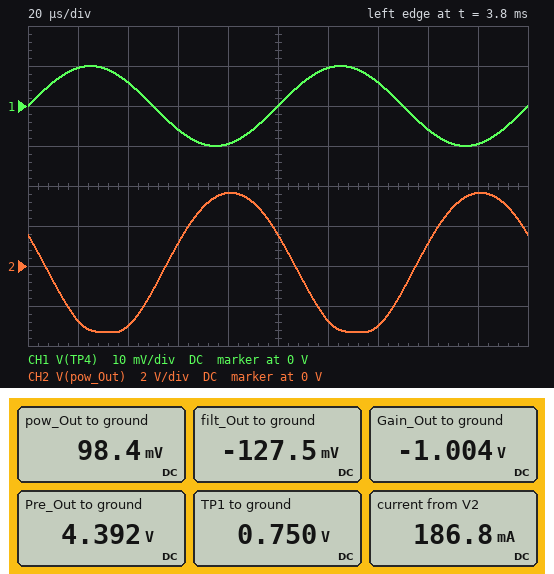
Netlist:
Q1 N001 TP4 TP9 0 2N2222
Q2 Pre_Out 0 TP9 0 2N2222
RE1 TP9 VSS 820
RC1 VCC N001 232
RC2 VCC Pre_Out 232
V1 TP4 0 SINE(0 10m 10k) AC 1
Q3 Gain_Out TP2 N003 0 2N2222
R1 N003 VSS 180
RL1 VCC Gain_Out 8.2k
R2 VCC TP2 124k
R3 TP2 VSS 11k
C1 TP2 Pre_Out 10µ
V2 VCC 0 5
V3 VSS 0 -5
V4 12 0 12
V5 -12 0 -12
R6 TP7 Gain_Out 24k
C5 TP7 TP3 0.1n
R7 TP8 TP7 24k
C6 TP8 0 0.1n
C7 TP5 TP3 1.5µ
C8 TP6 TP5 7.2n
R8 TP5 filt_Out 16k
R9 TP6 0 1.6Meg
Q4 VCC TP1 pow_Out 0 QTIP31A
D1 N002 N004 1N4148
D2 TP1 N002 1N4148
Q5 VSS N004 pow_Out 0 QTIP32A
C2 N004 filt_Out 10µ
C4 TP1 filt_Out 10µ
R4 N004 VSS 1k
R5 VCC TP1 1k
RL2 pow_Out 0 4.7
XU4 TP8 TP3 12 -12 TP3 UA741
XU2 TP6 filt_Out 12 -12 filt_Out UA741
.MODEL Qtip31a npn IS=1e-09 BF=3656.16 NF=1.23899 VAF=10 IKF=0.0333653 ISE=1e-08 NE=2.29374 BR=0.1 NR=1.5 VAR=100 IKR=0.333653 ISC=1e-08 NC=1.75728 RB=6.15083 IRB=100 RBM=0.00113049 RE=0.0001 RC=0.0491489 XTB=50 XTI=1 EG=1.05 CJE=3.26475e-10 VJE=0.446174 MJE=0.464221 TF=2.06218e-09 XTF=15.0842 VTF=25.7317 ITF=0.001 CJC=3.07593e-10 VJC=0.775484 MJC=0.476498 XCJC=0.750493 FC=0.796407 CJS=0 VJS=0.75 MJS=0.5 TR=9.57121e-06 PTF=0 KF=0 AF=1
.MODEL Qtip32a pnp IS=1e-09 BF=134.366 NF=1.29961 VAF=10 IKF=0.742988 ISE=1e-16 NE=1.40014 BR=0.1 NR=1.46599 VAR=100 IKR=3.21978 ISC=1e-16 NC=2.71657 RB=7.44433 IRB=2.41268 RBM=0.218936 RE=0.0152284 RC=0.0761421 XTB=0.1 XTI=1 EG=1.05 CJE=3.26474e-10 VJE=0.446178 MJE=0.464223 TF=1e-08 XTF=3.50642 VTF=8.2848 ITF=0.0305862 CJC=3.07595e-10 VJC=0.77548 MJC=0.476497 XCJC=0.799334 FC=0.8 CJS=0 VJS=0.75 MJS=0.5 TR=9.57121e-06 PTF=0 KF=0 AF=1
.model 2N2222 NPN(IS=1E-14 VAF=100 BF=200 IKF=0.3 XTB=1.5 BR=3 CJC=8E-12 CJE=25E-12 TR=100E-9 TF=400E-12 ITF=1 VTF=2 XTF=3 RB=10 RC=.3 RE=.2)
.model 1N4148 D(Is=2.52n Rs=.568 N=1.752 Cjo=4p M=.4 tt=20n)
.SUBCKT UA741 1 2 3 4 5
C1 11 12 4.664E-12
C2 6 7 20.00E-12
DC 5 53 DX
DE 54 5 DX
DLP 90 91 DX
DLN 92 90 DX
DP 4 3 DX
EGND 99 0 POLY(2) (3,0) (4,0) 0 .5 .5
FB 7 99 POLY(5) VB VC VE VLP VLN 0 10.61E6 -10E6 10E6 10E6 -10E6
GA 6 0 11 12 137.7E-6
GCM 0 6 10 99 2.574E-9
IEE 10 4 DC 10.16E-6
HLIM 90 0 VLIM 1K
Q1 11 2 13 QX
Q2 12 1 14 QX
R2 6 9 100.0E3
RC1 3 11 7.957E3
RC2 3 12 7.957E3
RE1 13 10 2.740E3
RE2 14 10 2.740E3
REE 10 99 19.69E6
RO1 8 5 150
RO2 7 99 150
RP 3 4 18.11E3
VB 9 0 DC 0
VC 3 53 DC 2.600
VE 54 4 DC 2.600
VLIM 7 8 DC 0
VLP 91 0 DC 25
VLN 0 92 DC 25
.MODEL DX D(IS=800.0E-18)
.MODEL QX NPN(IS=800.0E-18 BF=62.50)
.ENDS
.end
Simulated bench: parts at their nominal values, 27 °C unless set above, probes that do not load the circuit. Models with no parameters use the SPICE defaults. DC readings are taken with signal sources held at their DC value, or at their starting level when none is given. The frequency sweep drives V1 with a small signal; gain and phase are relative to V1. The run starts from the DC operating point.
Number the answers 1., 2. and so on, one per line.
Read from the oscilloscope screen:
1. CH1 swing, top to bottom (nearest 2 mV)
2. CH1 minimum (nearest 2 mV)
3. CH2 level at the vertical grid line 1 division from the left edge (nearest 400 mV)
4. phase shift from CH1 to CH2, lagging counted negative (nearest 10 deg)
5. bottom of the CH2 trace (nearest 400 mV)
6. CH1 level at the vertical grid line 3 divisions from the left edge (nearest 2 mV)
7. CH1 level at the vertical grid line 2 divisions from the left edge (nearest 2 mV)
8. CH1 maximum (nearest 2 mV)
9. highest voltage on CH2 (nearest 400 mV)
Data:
1. 20 mV
2. -10 mV
3. -2.8 V
4. 160 deg
5. -3.2 V
6. -6 mV
7. 6 mV
8. 10 mV
9. 3.6 V
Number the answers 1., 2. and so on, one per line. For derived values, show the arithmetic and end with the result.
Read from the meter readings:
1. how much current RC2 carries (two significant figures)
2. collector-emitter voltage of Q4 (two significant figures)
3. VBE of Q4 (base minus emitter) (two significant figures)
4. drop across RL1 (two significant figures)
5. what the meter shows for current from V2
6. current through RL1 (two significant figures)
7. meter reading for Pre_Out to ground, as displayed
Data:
1. (5 V - 4.392 V) / 232 Ω = 2.6 mA
2. 5 V - 98.4 mV = 4.9 V
3. 750 mV - 98.4 mV = 650 mV
4. 5 V - (-1.004 V) = 6.0 V
5. 186.8 mA
6. (5 V - (-1.004 V)) / 8.2 kΩ = 730 µA
7. 4.392 V
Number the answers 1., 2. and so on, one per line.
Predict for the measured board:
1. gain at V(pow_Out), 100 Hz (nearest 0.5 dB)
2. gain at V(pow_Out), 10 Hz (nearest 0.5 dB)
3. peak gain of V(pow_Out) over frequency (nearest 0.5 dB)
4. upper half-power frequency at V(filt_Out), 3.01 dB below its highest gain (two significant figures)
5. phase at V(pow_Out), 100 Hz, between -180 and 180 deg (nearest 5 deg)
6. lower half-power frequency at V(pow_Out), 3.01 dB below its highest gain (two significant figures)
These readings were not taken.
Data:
1. 51.5 dB
2. 40.0 dB
3. 52.0 dB
4. 37 kHz
5. -155 deg
6. 27 Hz
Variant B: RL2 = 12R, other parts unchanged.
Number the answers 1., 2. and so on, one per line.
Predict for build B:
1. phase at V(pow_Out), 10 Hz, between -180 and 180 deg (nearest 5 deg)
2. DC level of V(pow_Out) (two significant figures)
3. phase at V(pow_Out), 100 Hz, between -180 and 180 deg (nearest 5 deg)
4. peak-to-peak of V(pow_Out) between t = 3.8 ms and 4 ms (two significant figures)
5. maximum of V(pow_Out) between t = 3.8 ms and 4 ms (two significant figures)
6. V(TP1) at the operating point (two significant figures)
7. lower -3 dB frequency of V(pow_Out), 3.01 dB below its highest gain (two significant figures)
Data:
1. -20 deg
2. 130 mV
3. -160 deg
4. 7.2 V
5. 3.8 V
6. 780 mV
7. 22 Hz
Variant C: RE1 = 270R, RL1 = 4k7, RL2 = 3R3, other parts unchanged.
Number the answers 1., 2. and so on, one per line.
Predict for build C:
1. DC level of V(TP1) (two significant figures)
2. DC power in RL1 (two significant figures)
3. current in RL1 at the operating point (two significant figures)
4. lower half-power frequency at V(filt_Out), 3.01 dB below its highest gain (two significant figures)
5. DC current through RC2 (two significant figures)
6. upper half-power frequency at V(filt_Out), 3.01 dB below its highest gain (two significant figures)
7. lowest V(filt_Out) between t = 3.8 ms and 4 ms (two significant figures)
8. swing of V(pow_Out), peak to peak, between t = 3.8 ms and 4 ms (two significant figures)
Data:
1. 740 mV
2. 2.6 mW
3. 740 µA
4. 10 Hz
5. 7.9 mA
6. 40 kHz
7. -4.8 V
8. 7.3 V
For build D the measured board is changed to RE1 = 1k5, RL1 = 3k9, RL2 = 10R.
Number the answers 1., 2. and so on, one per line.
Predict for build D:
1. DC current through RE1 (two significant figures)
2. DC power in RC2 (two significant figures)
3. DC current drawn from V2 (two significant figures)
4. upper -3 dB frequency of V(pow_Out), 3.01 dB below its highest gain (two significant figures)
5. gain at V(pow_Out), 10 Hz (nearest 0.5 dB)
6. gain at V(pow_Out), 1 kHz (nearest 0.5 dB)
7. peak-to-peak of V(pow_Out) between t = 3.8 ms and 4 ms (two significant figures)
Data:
1. 2.9 mA
2. 480 µW
3. 180 mA
4. 40 kHz
5. 30.0 dB
6. 40.5 dB
7. 2.1 V
